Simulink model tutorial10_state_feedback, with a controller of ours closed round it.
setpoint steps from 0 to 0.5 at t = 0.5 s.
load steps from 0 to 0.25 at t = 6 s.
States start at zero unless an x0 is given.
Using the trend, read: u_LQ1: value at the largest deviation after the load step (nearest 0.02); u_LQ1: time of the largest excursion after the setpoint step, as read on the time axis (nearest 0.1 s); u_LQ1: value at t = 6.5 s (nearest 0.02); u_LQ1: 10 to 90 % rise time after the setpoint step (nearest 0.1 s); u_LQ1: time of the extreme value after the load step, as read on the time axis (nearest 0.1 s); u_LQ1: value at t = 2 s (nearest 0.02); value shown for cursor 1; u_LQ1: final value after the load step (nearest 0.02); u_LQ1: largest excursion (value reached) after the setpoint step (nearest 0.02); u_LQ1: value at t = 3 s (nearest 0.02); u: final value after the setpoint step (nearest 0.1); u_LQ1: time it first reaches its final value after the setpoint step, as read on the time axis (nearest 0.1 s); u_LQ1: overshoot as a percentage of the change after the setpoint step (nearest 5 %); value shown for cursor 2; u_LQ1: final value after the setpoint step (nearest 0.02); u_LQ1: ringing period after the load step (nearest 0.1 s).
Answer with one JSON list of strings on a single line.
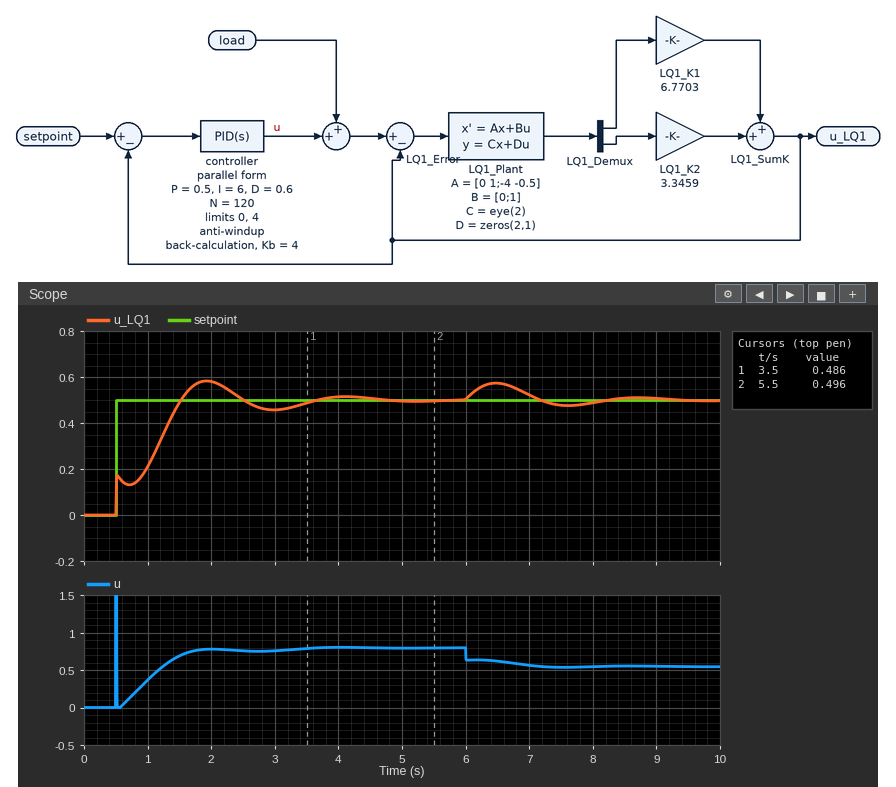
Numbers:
["0.58", "1.9 s", "0.58", "0.9 s", "6.5 s", "0.58", "0.486", "0.50", "0.58", "0.46", "0.8", "1.5 s", "15 %", "0.496", "0.50", "2.2 s"]
